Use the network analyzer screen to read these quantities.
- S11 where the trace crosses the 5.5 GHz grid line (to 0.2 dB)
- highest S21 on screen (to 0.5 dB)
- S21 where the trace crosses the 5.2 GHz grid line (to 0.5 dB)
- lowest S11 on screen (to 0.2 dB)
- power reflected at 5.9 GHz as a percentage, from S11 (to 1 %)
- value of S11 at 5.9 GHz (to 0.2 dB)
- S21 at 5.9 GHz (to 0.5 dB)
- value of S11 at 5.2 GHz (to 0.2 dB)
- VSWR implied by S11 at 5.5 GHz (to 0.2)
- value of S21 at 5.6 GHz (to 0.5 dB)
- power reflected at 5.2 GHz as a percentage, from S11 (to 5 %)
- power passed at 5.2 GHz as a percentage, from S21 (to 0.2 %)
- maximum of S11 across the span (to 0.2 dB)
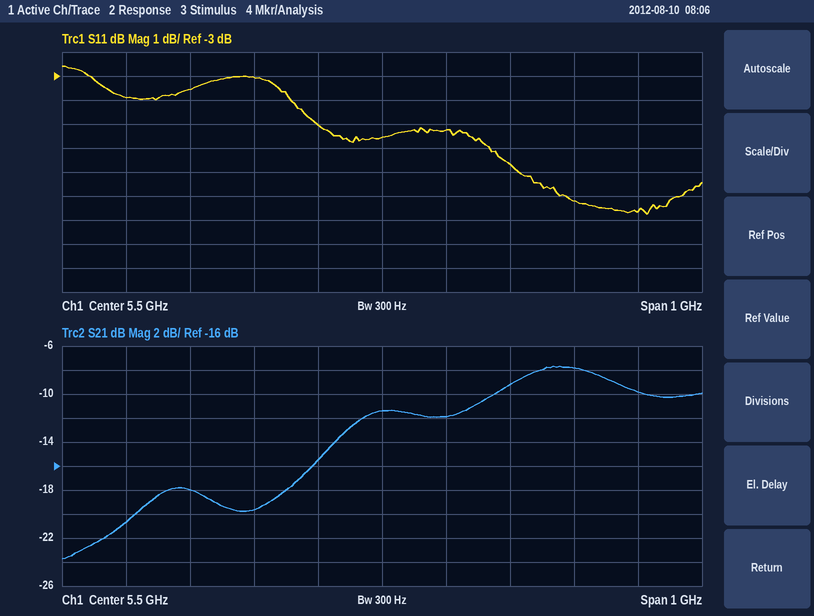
-5.6 dB
-7.5 dB
-18.0 dB
-8.8 dB
14 %
-8.6 dB
-10.0 dB
-3.6 dB
3.2
-12.0 dB
45 %
1.6 %
-2.6 dB
